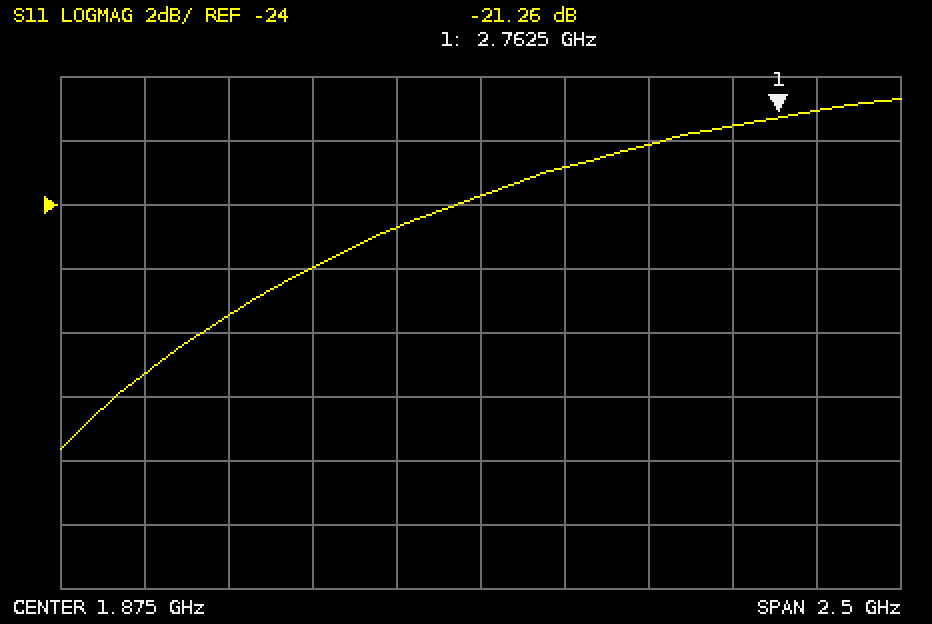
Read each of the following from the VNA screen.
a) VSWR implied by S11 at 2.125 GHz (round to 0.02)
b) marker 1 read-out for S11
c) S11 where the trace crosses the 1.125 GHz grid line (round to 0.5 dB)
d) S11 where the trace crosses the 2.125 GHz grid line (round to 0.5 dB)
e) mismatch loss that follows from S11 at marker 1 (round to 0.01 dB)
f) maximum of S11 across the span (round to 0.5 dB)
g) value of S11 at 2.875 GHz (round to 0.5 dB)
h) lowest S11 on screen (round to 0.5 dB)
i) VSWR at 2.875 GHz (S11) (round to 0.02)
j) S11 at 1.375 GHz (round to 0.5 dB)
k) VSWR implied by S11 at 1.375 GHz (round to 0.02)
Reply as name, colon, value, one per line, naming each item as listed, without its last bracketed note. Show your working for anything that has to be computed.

VSWR implied by S11 at 2.125 GHz: |Γ| = 10^(-23/20) = 0.0708; VSWR = (1 + 0.0708)/(1 − 0.0708) ≈ 1.15, so 1.16 to the nearest 0.02
marker 1 read-out for S11: -21.26 dB
S11 where the trace crosses the 1.125 GHz grid line: -27.5 dB
S11 where the trace crosses the 2.125 GHz grid line: -23.0 dB
mismatch loss that follows from S11 at marker 1: −10 log10(1 − 10^(-21.26/10)) ≈ 0.03 dB
maximum of S11 across the span: -20.5 dB
value of S11 at 2.875 GHz: -21.0 dB
lowest S11 on screen: -31.5 dB
VSWR at 2.875 GHz (S11): |Γ| = 10^(-21/20) = 0.0891; VSWR = (1 + 0.0891)/(1 − 0.0891) ≈ 1.20
S11 at 1.375 GHz: -26.0 dB
VSWR implied by S11 at 1.375 GHz: |Γ| = 10^(-26/20) = 0.0501; VSWR = (1 + 0.0501)/(1 − 0.0501) ≈ 1.11, so 1.10 to the nearest 0.02
